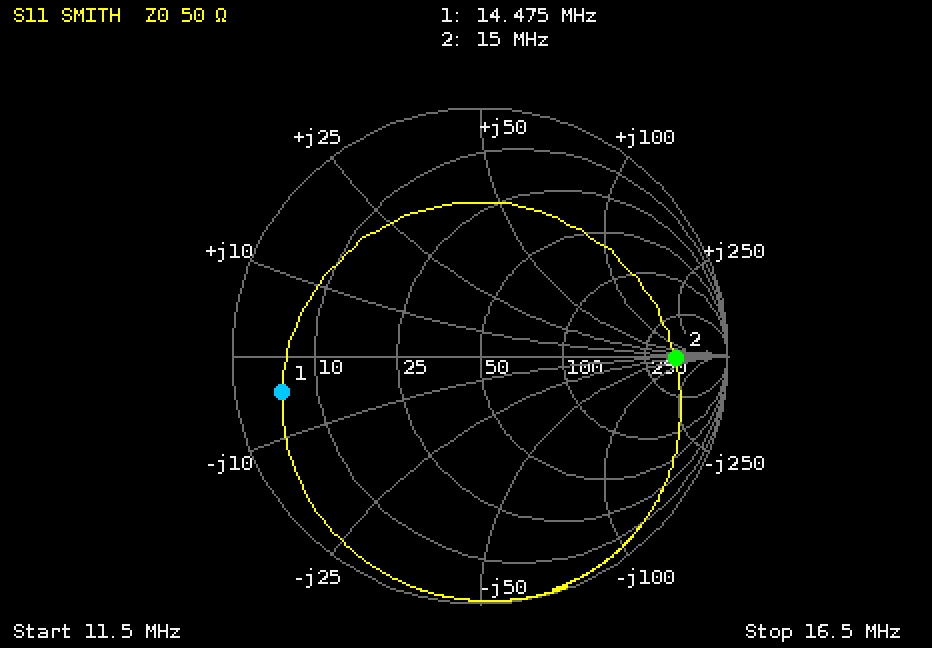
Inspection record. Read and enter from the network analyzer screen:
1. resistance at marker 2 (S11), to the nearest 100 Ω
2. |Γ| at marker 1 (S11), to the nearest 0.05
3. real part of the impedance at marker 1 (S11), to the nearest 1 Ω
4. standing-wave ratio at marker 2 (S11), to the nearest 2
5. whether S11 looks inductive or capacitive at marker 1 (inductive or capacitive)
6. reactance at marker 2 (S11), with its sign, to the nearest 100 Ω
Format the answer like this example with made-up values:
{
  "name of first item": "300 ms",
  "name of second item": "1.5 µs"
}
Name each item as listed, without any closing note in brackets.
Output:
{
  "resistance at marker 2 (S11), to the nearest 100 Ω": "400 Ω",
  "|Γ| at marker 1 (S11), to the nearest 0.05": "0.80",
  "real part of the impedance at marker 1 (S11), to the nearest 1 Ω": "5 Ω",
  "standing-wave ratio at marker 2 (S11), to the nearest 2": "8",
  "whether S11 looks inductive or capacitive at marker 1": "capacitive",
  "reactance at marker 2 (S11), with its sign, to the nearest 100 Ω": "0 Ω"
}
